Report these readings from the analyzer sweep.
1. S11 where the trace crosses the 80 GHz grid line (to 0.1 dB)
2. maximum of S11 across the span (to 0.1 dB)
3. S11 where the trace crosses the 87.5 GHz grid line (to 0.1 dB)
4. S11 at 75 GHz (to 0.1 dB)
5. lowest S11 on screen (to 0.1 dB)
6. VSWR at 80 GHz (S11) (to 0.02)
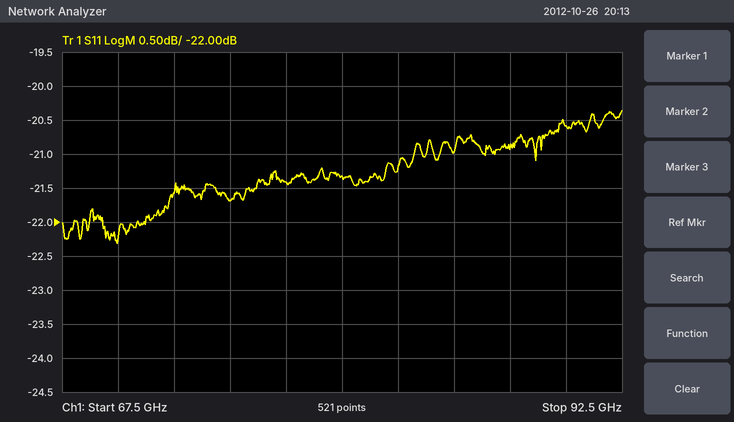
-21.3 dB
-20.4 dB
-20.9 dB
-21.7 dB
-22.3 dB
1.18
